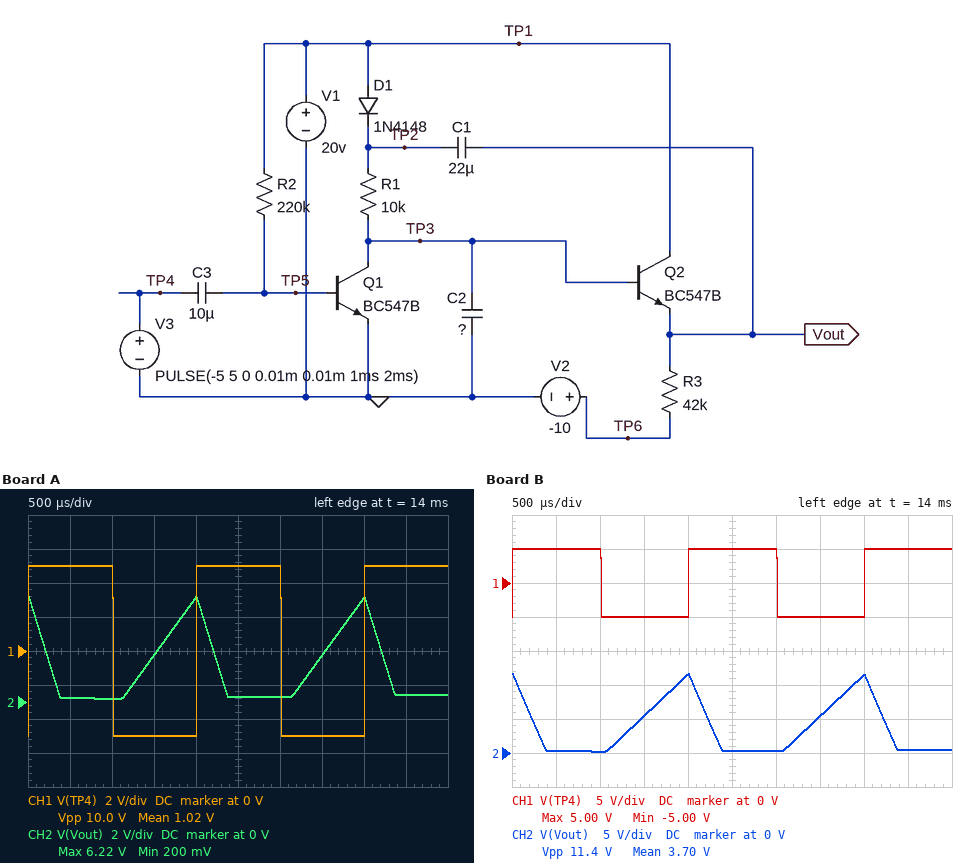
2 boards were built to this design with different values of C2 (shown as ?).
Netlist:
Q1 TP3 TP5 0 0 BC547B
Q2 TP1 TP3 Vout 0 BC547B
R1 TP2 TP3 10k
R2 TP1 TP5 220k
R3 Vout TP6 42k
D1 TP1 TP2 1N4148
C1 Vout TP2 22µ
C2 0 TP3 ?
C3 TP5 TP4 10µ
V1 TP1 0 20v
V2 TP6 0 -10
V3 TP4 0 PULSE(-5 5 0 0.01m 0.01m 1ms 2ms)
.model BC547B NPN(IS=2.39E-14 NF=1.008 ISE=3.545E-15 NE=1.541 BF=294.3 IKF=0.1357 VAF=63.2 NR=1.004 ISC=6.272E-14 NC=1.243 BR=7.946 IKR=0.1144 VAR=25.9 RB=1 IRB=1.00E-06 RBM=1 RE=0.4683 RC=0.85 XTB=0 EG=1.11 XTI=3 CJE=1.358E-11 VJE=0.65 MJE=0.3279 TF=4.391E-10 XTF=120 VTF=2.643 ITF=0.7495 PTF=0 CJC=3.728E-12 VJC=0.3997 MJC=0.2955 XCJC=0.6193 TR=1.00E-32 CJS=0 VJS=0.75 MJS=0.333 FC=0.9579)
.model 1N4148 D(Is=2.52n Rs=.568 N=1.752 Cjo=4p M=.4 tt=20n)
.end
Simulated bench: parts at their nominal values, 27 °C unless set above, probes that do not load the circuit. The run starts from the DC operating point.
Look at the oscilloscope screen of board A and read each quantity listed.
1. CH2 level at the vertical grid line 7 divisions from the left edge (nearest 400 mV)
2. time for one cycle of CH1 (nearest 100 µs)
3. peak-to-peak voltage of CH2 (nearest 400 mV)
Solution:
2.8 V
2.0 ms
6.0 V
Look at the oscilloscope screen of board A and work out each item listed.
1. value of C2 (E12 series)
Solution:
270 nF
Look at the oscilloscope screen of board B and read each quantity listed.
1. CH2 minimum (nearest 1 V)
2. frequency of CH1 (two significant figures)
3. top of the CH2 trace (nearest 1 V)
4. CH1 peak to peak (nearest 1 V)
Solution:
0 V
500 Hz
12 V
10 V
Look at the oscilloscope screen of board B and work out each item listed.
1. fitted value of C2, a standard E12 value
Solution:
150 nF
